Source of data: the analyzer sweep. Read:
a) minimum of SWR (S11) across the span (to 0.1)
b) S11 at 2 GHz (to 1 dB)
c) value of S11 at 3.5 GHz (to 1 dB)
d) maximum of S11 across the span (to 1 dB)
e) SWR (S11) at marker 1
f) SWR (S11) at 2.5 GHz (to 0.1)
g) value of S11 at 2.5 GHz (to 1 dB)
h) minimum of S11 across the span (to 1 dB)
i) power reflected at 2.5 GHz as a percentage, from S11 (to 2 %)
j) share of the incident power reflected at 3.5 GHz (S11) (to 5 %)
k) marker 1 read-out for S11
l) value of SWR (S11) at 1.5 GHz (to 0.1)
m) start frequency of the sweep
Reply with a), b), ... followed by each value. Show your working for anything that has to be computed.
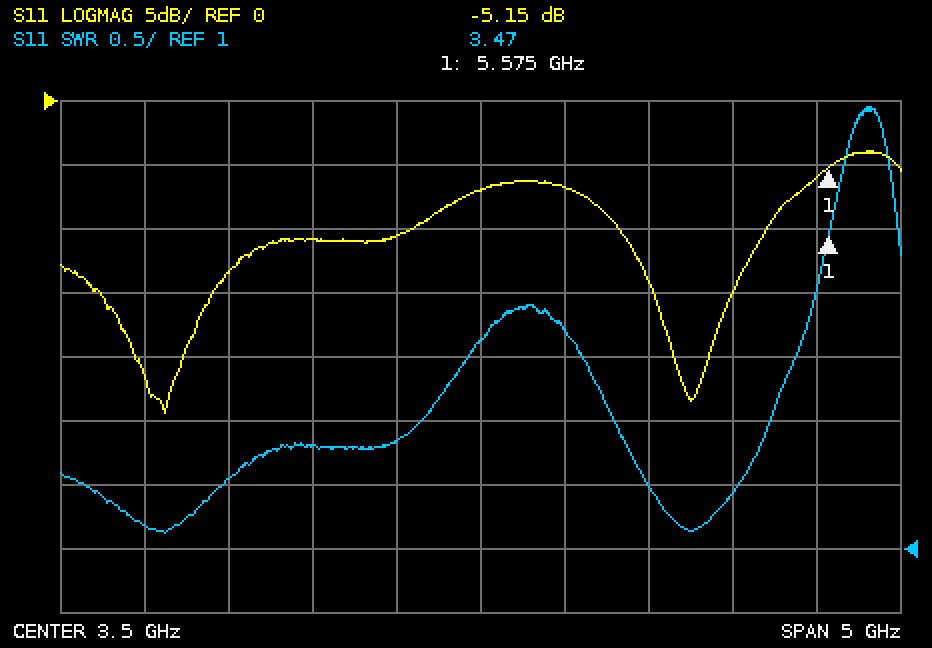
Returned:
a) 1.1
b) -13 dB
c) -7 dB
d) -4 dB
e) 3.47
f) 1.8
g) -11 dB
h) -24 dB
i) 10^(-11/10) ≈ 8 %
j) 10^(-7/10) ≈ 20 %
k) -5.15 dB
l) 1.2
m) 1 GHz
